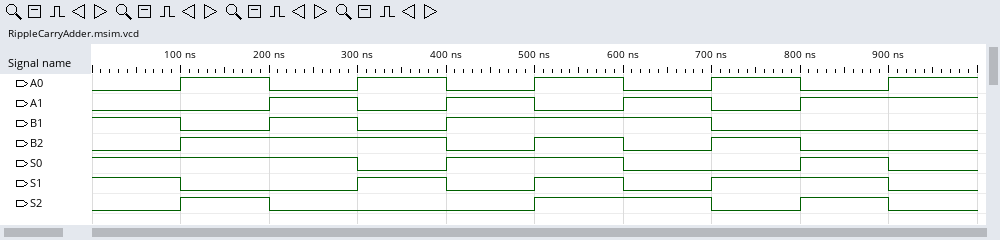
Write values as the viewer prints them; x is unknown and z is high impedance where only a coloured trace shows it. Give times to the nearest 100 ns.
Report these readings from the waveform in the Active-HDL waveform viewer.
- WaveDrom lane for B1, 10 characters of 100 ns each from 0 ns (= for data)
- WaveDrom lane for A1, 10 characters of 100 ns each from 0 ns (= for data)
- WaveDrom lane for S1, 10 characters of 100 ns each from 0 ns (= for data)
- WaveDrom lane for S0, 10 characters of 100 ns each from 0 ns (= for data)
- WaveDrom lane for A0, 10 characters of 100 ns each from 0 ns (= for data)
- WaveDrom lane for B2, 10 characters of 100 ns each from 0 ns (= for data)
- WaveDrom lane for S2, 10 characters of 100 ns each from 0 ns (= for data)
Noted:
{name: 'B1', wave: '10101..0..'}
{name: 'A1', wave: '0.1010101.'}
{name: 'S1', wave: '10.10101.0'}
{name: 'S0', wave: '1..01.0.10'}
{name: 'A0', wave: '0101010101'}
{name: 'B2', wave: '01..01010.'}
{name: 'S2', wave: '010..1.010'}
